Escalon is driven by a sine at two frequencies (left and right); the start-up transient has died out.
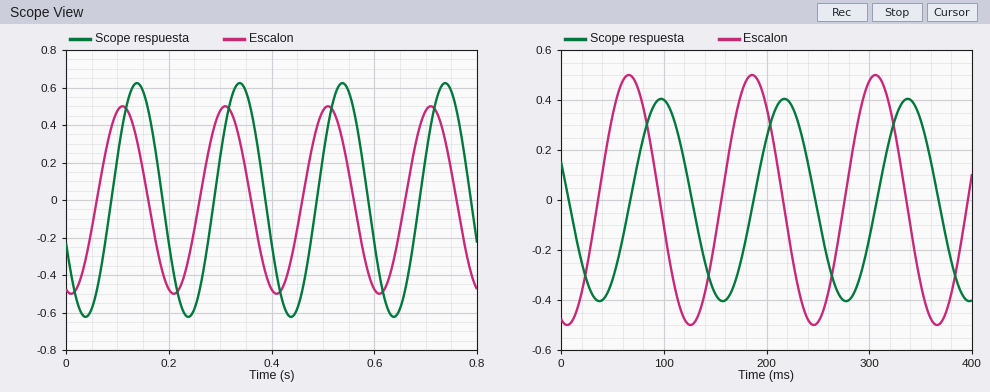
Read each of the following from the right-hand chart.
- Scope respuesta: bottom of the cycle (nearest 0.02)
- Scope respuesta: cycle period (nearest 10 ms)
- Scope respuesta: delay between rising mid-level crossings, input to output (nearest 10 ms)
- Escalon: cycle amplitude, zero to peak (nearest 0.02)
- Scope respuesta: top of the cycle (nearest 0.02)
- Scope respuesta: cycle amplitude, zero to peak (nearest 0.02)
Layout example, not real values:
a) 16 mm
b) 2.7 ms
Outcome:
a) -0.40
b) 120 ms
c) 30 ms
d) 0.50
e) 0.40
f) 0.40
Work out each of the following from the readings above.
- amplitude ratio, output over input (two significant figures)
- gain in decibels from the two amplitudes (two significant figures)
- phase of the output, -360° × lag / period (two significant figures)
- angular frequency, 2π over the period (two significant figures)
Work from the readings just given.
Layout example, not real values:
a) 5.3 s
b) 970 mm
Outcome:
a) 0.80
b) -1.9 dB
c) -90°
d) 0.052 rad/ms
